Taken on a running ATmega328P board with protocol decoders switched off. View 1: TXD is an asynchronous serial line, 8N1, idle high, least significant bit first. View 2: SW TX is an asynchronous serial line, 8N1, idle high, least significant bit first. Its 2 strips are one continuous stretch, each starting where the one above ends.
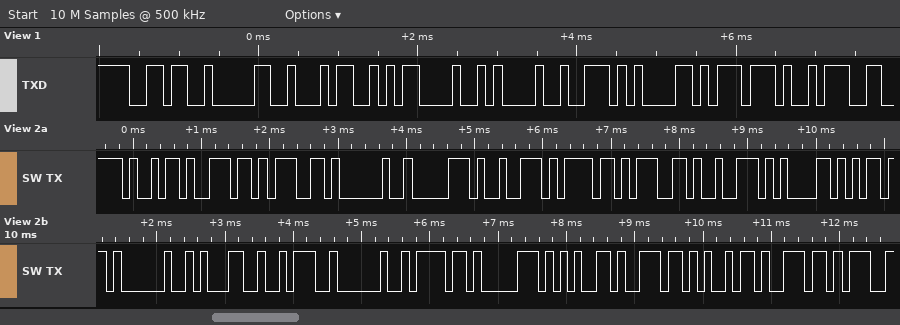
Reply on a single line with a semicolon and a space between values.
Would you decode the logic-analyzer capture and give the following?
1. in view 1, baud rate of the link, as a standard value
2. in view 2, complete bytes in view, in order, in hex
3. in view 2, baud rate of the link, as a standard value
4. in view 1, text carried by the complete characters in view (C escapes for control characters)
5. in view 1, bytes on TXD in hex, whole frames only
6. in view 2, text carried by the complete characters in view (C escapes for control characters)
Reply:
9600 baud; 0x69 0x6E 0x67 0x20 0x70 0x72 0x6F 0x67 0x72 0x61 0x6D 0x20 0x31 0x3A 0x20 0x6F 0x70 0x65 0x6E 0x69 0x6E; 9600 baud; "604\r\nraw:"; 0x36 0x30 0x34 0x0D 0x0A 0x72 0x61 0x77 0x3A; "ing program 1: openin"
